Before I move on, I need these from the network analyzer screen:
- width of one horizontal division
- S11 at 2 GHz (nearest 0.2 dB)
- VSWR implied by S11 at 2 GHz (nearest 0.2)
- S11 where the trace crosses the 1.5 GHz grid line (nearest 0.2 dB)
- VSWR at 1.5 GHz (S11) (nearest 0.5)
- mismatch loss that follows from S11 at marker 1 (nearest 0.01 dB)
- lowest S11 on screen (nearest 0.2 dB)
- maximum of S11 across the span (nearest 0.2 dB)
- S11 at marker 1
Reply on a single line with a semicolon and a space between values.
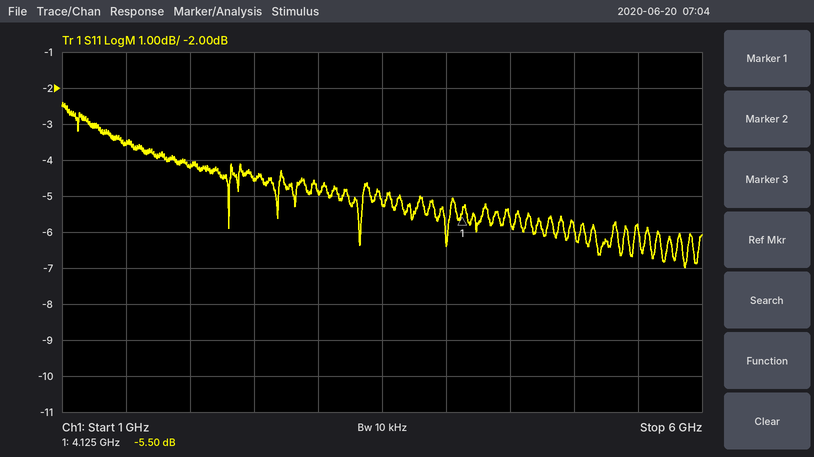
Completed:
500 MHz; -4.2 dB; 4.2; -3.6 dB; 5.0; 1.44 dB; -7.0 dB; -2.4 dB; -5.50 dB
